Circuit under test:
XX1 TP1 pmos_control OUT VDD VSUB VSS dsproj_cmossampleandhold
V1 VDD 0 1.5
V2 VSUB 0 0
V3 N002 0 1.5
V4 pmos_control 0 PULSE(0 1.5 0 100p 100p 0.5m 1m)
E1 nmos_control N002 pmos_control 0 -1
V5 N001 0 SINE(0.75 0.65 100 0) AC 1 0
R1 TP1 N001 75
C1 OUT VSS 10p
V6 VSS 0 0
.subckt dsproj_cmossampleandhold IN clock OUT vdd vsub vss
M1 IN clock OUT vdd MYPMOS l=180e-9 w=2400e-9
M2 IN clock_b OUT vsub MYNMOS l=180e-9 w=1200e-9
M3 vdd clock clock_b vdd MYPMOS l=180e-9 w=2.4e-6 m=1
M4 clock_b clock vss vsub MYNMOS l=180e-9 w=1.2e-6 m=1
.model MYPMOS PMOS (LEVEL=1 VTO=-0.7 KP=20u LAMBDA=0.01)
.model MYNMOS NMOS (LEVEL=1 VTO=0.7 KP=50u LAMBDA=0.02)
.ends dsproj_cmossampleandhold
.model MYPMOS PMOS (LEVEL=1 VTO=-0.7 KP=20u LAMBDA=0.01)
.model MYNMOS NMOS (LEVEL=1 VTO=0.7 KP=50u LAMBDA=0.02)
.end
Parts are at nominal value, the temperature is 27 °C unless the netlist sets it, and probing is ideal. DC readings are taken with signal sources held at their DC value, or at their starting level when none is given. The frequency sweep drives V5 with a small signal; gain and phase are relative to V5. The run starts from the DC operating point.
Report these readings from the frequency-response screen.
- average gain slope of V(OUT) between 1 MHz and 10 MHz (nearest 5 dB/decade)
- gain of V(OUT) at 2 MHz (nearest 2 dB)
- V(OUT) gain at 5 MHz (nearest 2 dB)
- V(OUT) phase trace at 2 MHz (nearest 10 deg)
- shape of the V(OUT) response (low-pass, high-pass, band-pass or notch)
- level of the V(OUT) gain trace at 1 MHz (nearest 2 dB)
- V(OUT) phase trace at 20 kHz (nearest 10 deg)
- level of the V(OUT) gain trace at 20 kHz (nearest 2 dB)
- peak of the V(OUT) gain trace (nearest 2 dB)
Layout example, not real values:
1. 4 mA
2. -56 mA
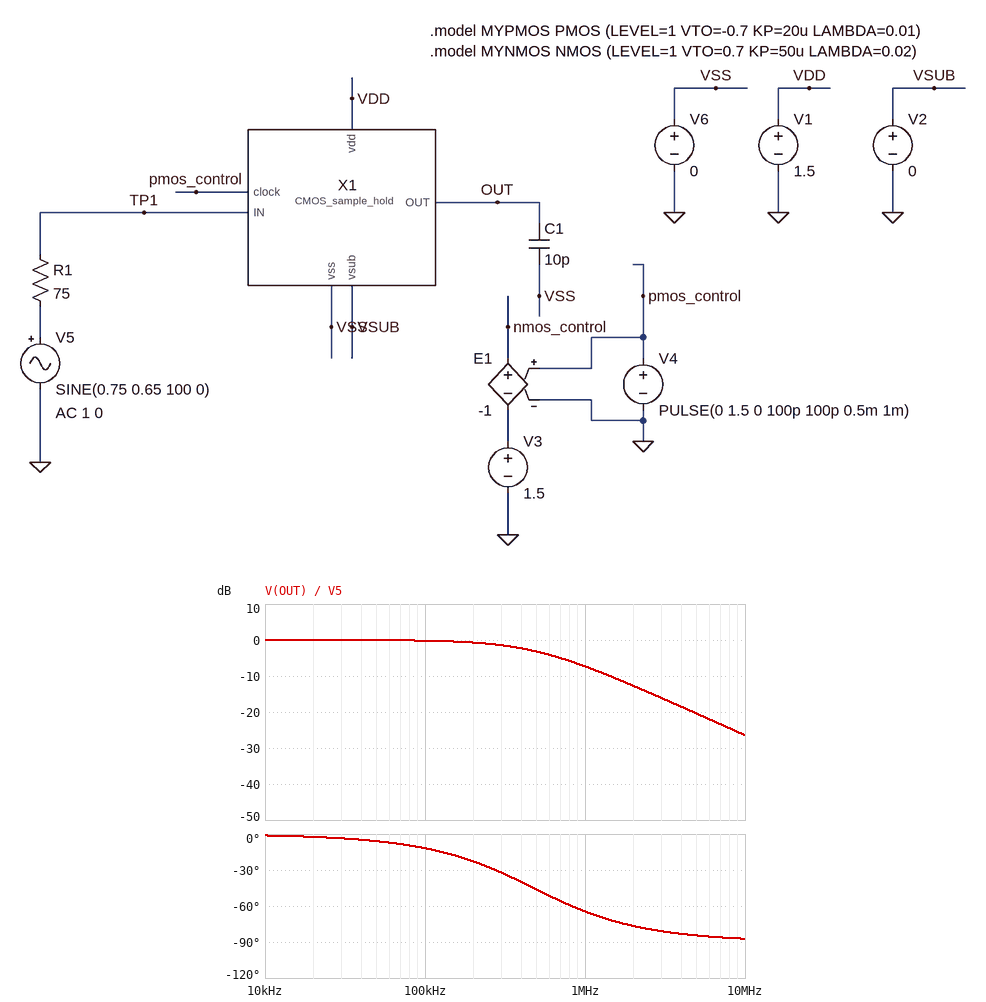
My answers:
1. -20 dB/decade
2. -12 dB
3. -20 dB
4. -80 deg
5. low-pass
6. -8 dB
7. 0 deg
8. 0 dB
9. 0 dB
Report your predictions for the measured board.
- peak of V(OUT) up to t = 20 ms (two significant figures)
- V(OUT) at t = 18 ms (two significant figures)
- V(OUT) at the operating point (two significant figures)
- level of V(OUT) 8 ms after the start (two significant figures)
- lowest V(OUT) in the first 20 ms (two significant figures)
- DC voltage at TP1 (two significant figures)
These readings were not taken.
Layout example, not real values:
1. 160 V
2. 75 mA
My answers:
1. 1.4 V
2. 130 mV
3. 750 mV
4. 130 mV
5. 100 mV
6. 750 mV
